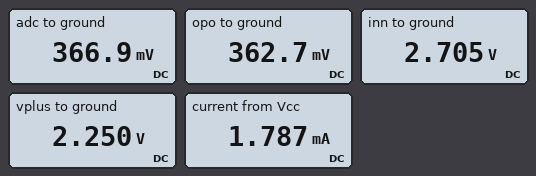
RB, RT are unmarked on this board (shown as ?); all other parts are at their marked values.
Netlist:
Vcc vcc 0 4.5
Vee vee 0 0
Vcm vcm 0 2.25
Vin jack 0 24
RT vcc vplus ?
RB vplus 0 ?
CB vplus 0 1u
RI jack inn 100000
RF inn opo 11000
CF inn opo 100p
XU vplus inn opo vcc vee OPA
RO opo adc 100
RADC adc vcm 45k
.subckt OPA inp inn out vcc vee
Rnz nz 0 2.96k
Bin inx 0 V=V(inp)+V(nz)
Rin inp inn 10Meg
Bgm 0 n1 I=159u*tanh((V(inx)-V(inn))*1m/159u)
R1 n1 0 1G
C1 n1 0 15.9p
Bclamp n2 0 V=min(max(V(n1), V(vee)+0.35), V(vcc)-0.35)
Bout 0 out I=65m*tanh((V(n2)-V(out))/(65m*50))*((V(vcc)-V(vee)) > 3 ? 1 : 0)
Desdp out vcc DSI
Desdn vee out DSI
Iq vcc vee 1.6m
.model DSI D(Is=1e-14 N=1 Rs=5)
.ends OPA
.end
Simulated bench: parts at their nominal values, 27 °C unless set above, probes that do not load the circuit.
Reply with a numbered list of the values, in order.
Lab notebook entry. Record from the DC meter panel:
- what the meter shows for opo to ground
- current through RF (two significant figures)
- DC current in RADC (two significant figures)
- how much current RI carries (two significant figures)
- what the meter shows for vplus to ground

1. 362.7 mV
2. 210 µA
3. 42 µA
4. 210 µA
5. 2.250 V
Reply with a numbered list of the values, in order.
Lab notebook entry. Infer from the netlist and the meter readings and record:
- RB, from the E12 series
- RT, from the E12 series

1. 12 kΩ
2. 12 kΩ
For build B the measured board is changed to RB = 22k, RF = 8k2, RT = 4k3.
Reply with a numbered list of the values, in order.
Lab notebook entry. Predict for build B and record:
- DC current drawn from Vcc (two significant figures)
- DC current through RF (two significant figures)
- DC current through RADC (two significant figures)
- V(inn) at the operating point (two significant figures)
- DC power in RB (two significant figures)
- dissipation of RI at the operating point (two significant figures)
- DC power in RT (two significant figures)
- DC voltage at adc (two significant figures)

1. 1.8 mA
2. 200 µA
3. 3.2 µA
4. 3.8 V
5. 640 µW
6. 4.1 mW
7. 130 µW
8. 2.1 V
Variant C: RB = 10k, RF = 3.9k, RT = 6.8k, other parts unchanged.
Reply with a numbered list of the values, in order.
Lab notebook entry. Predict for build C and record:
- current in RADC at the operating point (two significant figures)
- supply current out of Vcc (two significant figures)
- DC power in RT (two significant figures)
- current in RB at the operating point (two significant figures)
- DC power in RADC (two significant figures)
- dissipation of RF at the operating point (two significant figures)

1. 8.9 µA
2. 1.9 mA
3. 490 µW
4. 270 µA
5. 3.6 µW
6. 180 µW
